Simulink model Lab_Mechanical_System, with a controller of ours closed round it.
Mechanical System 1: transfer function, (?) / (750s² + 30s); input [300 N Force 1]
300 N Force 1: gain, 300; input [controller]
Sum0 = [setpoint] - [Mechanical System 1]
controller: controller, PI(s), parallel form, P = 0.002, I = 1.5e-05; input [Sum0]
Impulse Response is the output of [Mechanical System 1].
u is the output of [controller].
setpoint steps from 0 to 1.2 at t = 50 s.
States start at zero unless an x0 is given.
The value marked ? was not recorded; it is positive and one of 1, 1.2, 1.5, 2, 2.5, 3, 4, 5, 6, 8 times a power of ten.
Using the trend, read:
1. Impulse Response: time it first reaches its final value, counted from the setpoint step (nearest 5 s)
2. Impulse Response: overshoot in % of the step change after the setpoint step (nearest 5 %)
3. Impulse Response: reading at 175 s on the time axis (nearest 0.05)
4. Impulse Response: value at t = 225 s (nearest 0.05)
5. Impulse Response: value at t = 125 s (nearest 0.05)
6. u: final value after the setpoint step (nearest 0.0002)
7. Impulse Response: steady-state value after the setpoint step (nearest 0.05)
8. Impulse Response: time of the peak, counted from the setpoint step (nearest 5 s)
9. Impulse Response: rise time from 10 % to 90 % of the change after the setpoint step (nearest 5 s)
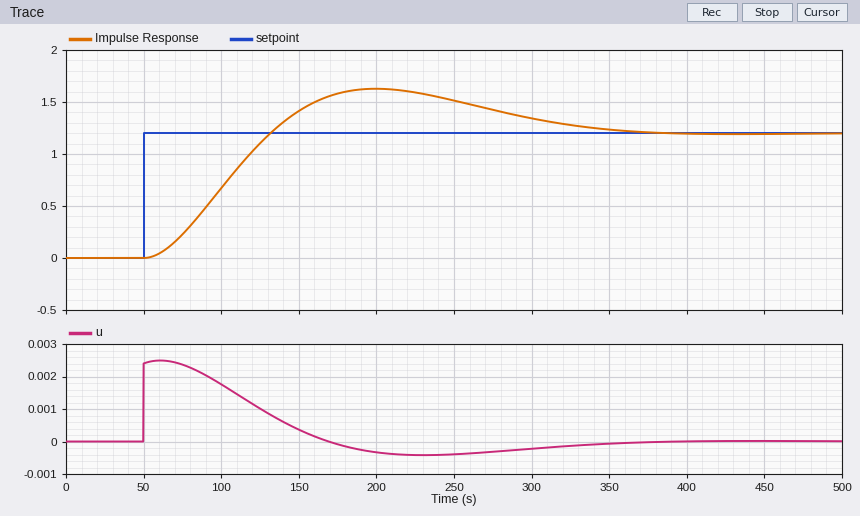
80 s
35 %
1.60
1.60
1.10
0.0000
1.20
150 s
55 s
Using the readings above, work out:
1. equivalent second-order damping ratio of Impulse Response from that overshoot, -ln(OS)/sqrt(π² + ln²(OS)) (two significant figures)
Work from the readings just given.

0.32
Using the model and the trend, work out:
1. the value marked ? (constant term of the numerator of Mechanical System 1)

1
